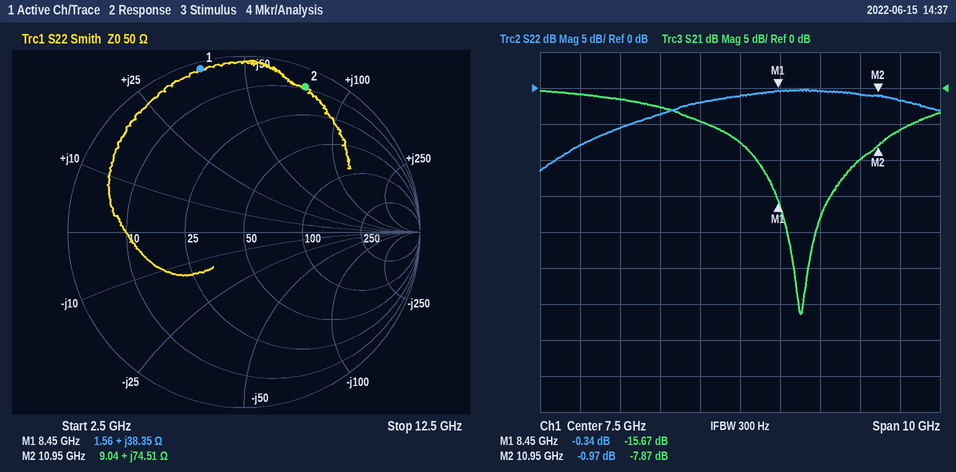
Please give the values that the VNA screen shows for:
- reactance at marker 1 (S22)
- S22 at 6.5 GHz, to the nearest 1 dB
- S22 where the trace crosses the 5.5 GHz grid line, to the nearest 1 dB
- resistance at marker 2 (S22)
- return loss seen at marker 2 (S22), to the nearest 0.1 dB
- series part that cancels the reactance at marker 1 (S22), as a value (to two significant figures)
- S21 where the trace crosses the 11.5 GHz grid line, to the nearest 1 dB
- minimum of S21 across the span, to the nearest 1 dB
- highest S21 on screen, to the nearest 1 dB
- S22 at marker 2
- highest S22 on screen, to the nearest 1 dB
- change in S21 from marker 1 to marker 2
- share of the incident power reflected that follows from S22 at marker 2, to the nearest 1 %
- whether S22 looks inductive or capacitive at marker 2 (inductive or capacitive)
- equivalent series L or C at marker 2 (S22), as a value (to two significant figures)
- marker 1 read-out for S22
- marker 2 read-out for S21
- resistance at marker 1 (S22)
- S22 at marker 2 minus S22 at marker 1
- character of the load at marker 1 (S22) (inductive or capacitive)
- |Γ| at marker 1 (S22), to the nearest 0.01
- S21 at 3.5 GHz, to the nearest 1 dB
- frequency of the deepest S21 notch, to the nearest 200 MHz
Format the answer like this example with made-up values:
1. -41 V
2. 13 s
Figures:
1. +38.35 Ω
2. -2 dB
3. -4 dB
4. 9.04 Ω
5. 1.0 dB
6. 490 fF
7. -6 dB
8. -31 dB
9. 0 dB
10. -0.97 dB
11. 0 dB
12. 7.80 dB
13. 80 %
14. inductive
15. 1.1 nH
16. -0.34 dB
17. -7.87 dB
18. 1.56 Ω
19. -0.63 dB
20. inductive
21. 0.96
22. -1 dB
23. 9.0 GHz
